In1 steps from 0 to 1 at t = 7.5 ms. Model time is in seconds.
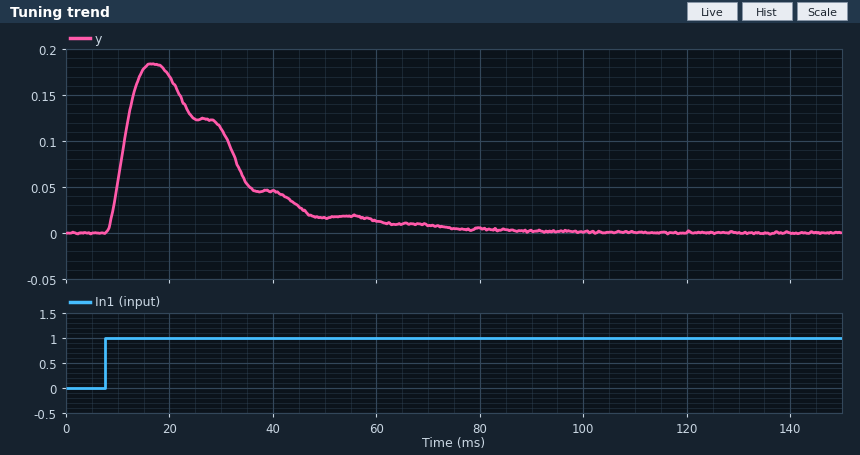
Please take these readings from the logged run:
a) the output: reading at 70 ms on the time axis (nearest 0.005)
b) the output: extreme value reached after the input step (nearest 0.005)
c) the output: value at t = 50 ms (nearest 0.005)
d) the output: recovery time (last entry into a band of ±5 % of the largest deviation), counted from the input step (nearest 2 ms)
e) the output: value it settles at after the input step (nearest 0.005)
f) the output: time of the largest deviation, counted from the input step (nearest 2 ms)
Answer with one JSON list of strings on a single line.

["0.010", "0.185", "0.015", "62 ms", "0.000", "10 ms"]
